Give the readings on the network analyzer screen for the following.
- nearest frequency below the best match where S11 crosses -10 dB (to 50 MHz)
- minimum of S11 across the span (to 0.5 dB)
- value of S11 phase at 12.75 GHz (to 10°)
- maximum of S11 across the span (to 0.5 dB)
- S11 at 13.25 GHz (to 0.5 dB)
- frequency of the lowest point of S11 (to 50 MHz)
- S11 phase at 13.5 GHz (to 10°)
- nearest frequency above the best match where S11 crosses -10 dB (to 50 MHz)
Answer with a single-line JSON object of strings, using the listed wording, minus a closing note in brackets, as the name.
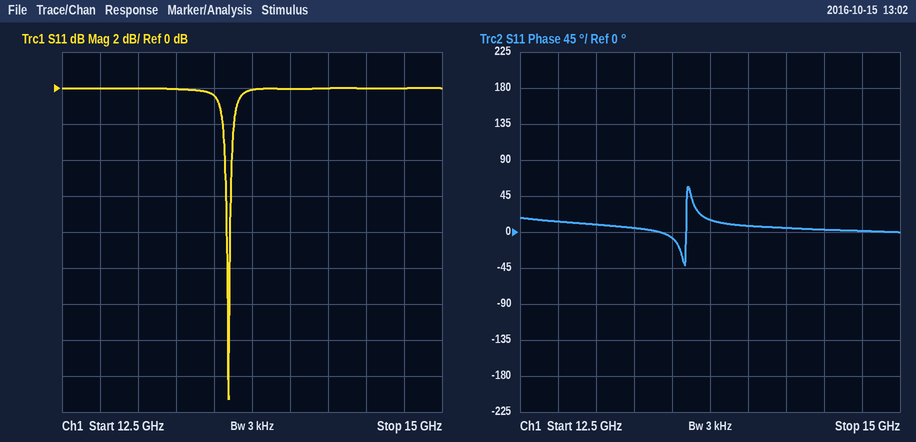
{"nearest frequency below the best match where S11 crosses -10 dB": "13.60 GHz", "minimum of S11 across the span": "-17.5 dB", "value of S11 phase at 12.75 GHz": "10°", "maximum of S11 across the span": "0.0 dB", "S11 at 13.25 GHz": "0.0 dB", "frequency of the lowest point of S11": "13.60 GHz", "S11 phase at 13.5 GHz": "-10°", "nearest frequency above the best match where S11 crosses -10 dB": "13.60 GHz"}
